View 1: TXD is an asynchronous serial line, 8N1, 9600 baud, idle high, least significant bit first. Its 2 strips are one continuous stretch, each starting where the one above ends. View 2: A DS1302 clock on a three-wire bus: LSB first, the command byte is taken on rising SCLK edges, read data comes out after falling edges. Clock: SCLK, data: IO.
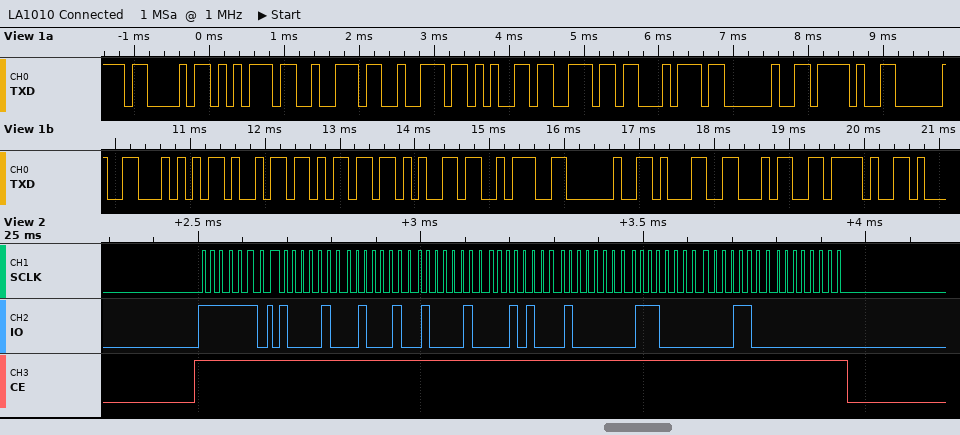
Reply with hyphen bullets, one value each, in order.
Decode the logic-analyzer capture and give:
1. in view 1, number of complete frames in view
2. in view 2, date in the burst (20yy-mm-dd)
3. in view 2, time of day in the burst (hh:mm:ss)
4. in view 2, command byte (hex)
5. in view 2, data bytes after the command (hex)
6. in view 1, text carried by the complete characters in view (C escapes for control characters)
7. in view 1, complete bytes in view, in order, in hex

- 19
- 2018-01-14
- 21:22:21
- 0xBF
- 21 22 21 14 01 07 18 00
- "Current / Time: 14/"
- 43 75 72 72 65 6E 74 20 2F 20 54 69 6D 65 3A 20 31 34 2F
